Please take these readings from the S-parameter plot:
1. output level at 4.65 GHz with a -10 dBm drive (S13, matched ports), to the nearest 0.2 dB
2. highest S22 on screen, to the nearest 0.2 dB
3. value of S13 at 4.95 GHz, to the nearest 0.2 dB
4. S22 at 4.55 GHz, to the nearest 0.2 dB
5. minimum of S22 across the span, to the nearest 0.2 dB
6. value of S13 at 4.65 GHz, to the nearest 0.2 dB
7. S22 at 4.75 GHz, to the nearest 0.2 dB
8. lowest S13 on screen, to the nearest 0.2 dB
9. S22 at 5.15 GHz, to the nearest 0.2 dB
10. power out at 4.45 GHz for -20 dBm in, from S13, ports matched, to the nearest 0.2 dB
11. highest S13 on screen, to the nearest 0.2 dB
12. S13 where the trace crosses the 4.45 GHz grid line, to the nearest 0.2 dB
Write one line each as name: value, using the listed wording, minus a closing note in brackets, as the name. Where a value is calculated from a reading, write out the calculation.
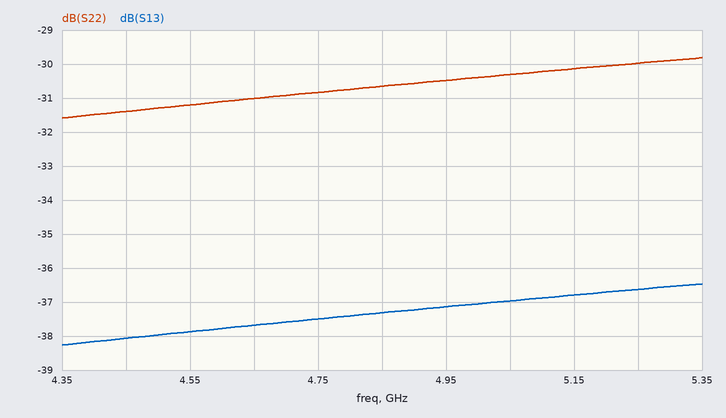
output level at 4.65 GHz with a -10 dBm drive (S13, matched ports), to the nearest 0.2 dB: -10 dBm + (-37.6 dB) = -47.6 dBm
highest S22 on screen, to the nearest 0.2 dB: -29.8 dB
value of S13 at 4.95 GHz, to the nearest 0.2 dB: -37.2 dB
S22 at 4.55 GHz, to the nearest 0.2 dB: -31.2 dB
minimum of S22 across the span, to the nearest 0.2 dB: -31.6 dB
value of S13 at 4.65 GHz, to the nearest 0.2 dB: -37.6 dB
S22 at 4.75 GHz, to the nearest 0.2 dB: -30.8 dB
lowest S13 on screen, to the nearest 0.2 dB: -38.2 dB
S22 at 5.15 GHz, to the nearest 0.2 dB: -30.2 dB
power out at 4.45 GHz for -20 dBm in, from S13, ports matched, to the nearest 0.2 dB: -20 dBm + (-38.0 dB) = -58.0 dBm
highest S13 on screen, to the nearest 0.2 dB: -36.4 dB
S13 where the trace crosses the 4.45 GHz grid line, to the nearest 0.2 dB: -38.0 dB
